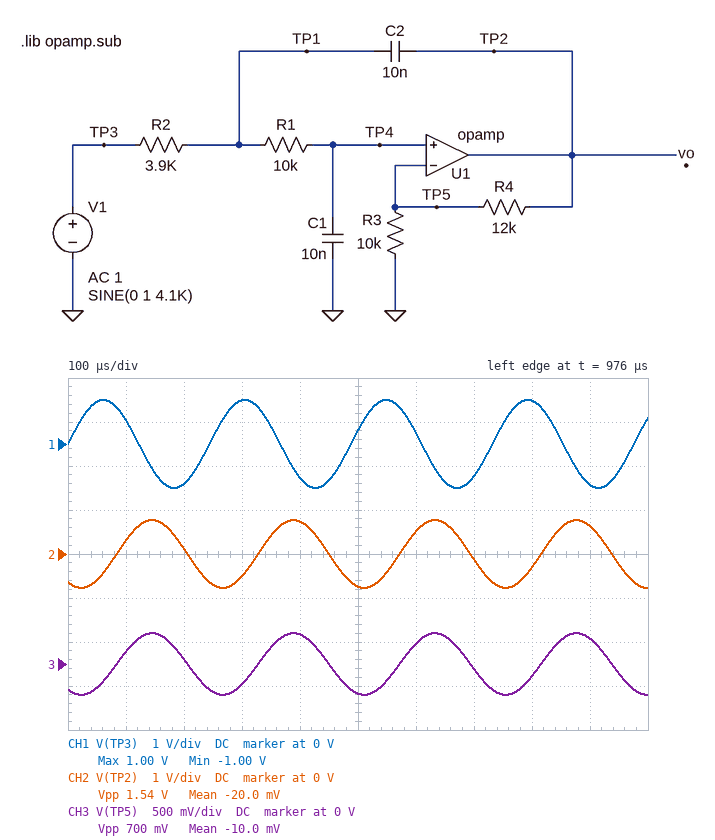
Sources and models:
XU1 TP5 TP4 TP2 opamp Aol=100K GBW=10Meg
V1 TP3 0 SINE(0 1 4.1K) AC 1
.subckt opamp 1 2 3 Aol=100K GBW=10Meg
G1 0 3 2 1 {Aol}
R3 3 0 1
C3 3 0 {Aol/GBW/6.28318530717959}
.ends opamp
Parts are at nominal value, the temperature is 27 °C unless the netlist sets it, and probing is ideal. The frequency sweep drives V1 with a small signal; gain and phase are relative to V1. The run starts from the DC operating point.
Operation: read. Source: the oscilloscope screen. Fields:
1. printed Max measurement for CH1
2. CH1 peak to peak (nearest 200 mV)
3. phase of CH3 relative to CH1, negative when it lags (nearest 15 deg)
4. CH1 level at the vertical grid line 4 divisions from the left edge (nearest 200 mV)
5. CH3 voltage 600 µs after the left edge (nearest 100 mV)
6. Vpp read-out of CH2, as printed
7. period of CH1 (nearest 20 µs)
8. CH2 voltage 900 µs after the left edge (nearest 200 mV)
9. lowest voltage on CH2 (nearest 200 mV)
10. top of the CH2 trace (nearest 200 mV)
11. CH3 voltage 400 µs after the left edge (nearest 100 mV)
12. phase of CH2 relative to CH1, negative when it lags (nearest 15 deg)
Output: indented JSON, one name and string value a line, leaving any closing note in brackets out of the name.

{
  "printed Max measurement for CH1": "1.00 V",
  "CH1 peak to peak": "2.0 V",
  "phase of CH3 relative to CH1, negative when it lags": "-120 deg",
  "CH1 level at the vertical grid line 4 divisions from the left edge": "-800 mV",
  "CH3 voltage 600 µs after the left edge": "200 mV",
  "Vpp read-out of CH2, as printed": "1.54 V",
  "period of CH1": "240 µs",
  "CH2 voltage 900 µs after the left edge": "600 mV",
  "lowest voltage on CH2": "-800 mV",
  "top of the CH2 trace": "800 mV",
  "CH3 voltage 400 µs after the left edge": "300 mV",
  "phase of CH2 relative to CH1, negative when it lags": "-120 deg"
}
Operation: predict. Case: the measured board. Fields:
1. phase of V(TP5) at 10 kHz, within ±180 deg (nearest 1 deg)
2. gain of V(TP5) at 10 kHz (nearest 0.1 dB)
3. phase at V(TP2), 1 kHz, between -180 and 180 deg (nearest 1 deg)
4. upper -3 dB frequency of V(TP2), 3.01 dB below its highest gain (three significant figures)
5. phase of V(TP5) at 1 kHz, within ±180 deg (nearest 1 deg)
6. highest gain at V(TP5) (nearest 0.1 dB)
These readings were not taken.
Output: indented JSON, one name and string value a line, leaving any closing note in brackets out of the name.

{
  "phase of V(TP5) at 10 kHz, within ±180 deg": "-158 deg",
  "gain of V(TP5) at 10 kHz": "-23.8 dB",
  "phase at V(TP2), 1 kHz, between -180 and 180 deg": "-34 deg",
  "upper -3 dB frequency of V(TP2), 3.01 dB below its highest gain": "2.44 kHz",
  "phase of V(TP5) at 1 kHz, within ±180 deg": "-34 deg",
  "highest gain at V(TP5)": "0 dB"
}
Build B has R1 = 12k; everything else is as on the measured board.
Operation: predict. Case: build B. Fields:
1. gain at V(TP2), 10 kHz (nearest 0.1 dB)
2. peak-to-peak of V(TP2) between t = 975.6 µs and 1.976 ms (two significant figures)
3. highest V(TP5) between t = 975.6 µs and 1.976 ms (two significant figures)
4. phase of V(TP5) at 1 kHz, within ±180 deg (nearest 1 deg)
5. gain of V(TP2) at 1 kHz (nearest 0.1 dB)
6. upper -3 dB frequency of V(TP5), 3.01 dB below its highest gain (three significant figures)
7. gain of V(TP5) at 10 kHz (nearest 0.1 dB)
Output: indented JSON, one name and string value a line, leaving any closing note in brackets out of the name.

{
  "gain at V(TP2), 10 kHz": "-18.7 dB",
  "peak-to-peak of V(TP2) between t = 975.6 µs and 1.976 ms": "1.2 V",
  "highest V(TP5) between t = 975.6 µs and 1.976 ms": "280 mV",
  "phase of V(TP5) at 1 kHz, within ±180 deg": "-41 deg",
  "gain of V(TP2) at 1 kHz": "6.2 dB",
  "upper -3 dB frequency of V(TP5), 3.01 dB below its highest gain": "1.96 kHz",
  "gain of V(TP5) at 10 kHz": "-25.5 dB"
}
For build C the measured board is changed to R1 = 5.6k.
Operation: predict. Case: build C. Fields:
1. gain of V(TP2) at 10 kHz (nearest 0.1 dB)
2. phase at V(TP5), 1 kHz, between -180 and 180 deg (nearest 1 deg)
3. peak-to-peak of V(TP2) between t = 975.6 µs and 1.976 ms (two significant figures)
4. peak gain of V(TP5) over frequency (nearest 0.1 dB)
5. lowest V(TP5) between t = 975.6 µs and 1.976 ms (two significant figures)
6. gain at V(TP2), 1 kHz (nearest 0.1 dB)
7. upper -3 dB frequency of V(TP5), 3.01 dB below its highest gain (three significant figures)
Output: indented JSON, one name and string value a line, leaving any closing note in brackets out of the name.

{
  "gain of V(TP2) at 10 kHz": "-11.4 dB",
  "phase at V(TP5), 1 kHz, between -180 and 180 deg": "-18 deg",
  "peak-to-peak of V(TP2) between t = 975.6 µs and 1.976 ms": "3.3 V",
  "peak gain of V(TP5) over frequency": "1.1 dB",
  "lowest V(TP5) between t = 975.6 µs and 1.976 ms": "-760 mV",
  "gain at V(TP2), 1 kHz": "7.2 dB",
  "upper -3 dB frequency of V(TP5), 3.01 dB below its highest gain": "3.96 kHz"
}
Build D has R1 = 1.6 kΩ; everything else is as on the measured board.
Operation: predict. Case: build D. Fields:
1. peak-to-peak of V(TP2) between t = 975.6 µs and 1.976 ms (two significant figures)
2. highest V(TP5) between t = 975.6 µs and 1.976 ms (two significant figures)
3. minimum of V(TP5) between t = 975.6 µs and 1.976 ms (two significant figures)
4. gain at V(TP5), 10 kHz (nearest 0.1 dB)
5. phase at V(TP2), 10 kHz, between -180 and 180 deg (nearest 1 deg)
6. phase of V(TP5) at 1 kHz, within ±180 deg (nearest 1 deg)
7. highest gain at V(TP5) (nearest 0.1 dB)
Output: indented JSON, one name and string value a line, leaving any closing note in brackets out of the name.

{
  "peak-to-peak of V(TP2) between t = 975.6 µs and 1.976 ms": "7.1 V",
  "highest V(TP5) between t = 975.6 µs and 1.976 ms": "1.6 V",
  "minimum of V(TP5) between t = 975.6 µs and 1.976 ms": "-1.6 V",
  "gain at V(TP5), 10 kHz": "-3.9 dB",
  "phase at V(TP2), 10 kHz, between -180 and 180 deg": "-161 deg",
  "phase of V(TP5) at 1 kHz, within ±180 deg": "-3 deg",
  "highest gain at V(TP5)": "9.8 dB"
}
